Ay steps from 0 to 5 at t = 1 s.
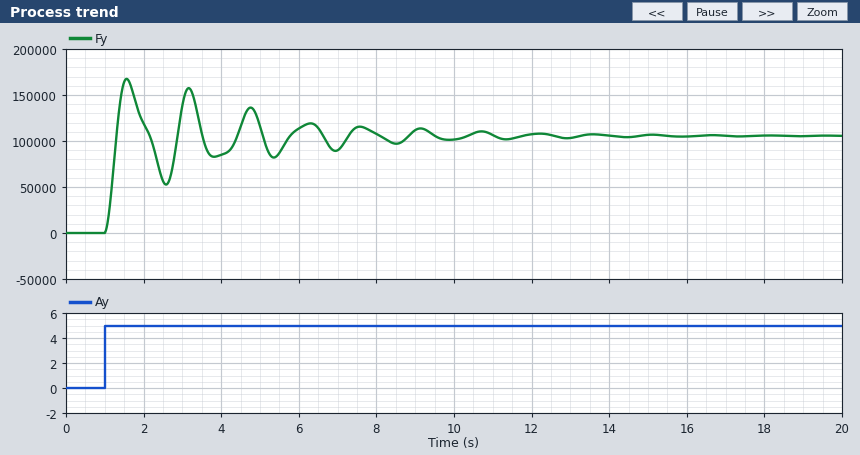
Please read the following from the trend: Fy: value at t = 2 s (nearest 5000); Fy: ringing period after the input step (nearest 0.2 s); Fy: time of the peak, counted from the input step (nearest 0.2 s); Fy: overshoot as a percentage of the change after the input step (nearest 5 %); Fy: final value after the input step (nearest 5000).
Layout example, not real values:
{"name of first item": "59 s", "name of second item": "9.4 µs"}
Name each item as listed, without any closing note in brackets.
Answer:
{"Fy: value at t = 2 s": "120000", "Fy: ringing period after the input step": "1.6 s", "Fy: time of the peak, counted from the input step": "0.6 s", "Fy: overshoot as a percentage of the change after the input step": "60 %", "Fy: final value after the input step": "105000"}
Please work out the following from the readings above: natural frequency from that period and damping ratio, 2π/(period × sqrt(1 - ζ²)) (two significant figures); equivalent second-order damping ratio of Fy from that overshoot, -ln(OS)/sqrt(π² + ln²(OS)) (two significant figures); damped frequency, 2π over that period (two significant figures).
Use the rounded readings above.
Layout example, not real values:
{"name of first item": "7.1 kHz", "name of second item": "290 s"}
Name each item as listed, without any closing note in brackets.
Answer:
{"natural frequency from that period and damping ratio, 2π/(period × sqrt(1 - ζ²))": "4.0 rad/s", "equivalent second-order damping ratio of Fy from that overshoot, -ln(OS)/sqrt(π² + ln²(OS))": "0.16", "damped frequency, 2π over that period": "3.9 rad/s"}
